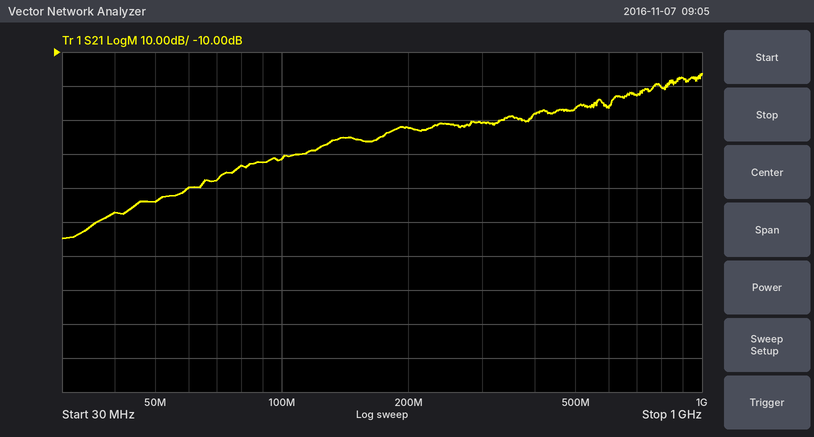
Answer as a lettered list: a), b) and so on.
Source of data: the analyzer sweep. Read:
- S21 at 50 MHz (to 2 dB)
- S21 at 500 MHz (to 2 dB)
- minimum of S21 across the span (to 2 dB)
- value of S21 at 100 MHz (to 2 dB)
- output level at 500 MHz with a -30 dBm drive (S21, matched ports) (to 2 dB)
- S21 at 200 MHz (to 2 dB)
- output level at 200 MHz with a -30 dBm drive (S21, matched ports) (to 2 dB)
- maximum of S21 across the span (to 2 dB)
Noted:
a) -54 dB
b) -26 dB
c) -64 dB
d) -42 dB
e) -56 dBm
f) -32 dB
g) -62 dBm
h) -16 dB
